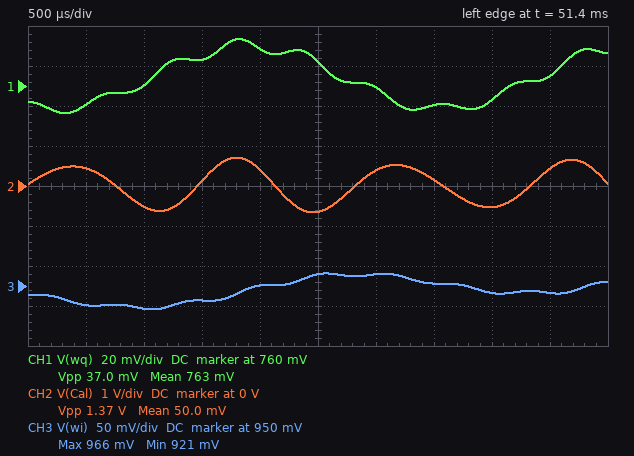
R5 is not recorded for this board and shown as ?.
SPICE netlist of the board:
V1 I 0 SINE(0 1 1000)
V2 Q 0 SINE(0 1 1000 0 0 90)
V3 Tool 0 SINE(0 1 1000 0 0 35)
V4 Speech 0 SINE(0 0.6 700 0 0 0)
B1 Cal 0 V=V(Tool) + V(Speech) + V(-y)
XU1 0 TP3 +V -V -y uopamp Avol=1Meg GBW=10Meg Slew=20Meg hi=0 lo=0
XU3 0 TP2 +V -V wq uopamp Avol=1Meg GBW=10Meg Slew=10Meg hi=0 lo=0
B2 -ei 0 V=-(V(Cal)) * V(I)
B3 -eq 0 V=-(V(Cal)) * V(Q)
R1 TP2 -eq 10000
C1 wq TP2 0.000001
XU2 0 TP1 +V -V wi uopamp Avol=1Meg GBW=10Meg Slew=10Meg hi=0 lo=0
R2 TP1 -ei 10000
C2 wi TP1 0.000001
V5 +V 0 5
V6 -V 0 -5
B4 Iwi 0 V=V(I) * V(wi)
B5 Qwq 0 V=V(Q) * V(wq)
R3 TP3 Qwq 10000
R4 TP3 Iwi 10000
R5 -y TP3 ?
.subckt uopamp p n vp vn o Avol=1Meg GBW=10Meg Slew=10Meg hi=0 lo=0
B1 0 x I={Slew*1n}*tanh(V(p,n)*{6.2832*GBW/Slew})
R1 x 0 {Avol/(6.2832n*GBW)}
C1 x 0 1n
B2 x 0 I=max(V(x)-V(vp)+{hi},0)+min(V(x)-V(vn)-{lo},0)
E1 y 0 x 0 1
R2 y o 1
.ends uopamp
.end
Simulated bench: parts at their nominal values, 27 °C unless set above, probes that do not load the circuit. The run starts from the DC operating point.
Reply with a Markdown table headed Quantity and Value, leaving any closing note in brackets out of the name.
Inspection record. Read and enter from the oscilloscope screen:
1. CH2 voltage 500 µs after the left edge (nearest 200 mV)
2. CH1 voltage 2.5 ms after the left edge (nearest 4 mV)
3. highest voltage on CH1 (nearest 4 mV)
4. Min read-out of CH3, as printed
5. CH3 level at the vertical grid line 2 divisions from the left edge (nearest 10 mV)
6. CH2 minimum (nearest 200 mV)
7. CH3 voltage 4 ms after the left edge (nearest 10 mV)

| Quantity | Value |
|---|---|
| CH2 voltage 500 µs after the left edge | 400 mV |
| CH1 voltage 2.5 ms after the left edge | 772 mV |
| highest voltage on CH1 | 784 mV |
| Min read-out of CH3, as printed | 921 mV |
| CH3 level at the vertical grid line 2 divisions from the left edge | 920 mV |
| CH2 minimum | -600 mV |
| CH3 voltage 4 ms after the left edge | 940 mV |
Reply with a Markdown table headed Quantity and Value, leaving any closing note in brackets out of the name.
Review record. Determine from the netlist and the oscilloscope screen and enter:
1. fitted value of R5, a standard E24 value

| Quantity | Value |
|---|---|
| fitted value of R5, a standard E24 value | 7.5 kΩ |
